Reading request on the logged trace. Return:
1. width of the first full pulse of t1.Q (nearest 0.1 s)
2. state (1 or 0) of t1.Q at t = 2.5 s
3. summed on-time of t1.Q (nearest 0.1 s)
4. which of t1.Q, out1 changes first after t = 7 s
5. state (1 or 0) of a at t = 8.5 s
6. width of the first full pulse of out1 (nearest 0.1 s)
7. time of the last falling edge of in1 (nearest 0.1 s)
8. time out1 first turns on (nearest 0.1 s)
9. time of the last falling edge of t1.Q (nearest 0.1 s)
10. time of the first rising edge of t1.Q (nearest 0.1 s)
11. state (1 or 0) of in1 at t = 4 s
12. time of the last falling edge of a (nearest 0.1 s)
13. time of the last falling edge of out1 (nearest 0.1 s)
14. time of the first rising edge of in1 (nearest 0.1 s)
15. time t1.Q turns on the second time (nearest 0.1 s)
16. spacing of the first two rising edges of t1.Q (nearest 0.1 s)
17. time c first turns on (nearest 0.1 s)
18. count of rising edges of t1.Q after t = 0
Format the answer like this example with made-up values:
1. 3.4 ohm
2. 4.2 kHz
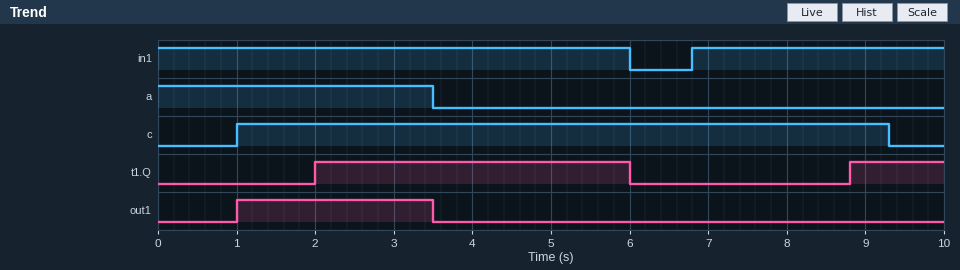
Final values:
1. 4.0 s
2. 1
3. 5.2 s
4. t1.Q
5. 0
6. 2.5 s
7. 6.0 s
8. 1.0 s
9. 6.0 s
10. 2.0 s
11. 1
12. 3.5 s
13. 3.5 s
14. 6.8 s
15. 8.8 s
16. 6.8 s
17. 1.0 s
18. 2
